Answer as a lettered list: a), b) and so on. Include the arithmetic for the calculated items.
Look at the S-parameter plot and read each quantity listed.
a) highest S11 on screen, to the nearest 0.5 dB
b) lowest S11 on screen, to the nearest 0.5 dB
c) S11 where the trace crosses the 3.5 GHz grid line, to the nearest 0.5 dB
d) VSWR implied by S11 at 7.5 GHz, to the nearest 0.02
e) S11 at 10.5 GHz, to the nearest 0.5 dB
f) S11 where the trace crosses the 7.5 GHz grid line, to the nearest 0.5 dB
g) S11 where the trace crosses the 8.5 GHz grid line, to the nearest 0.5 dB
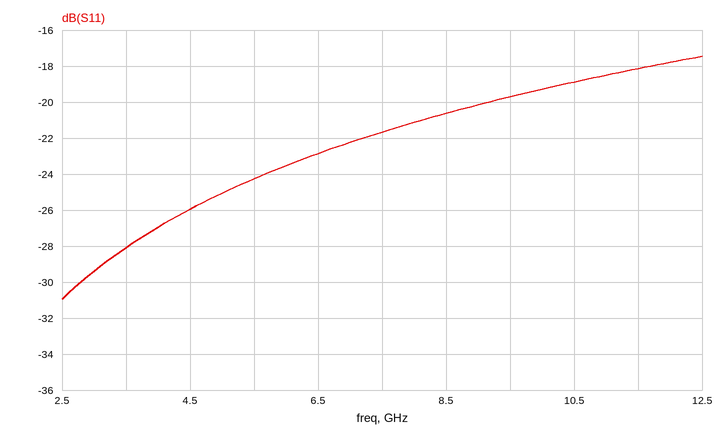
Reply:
a) -17.5 dB
b) -31.0 dB
c) -28.0 dB
d) |Γ| = 10^(-21.5/20) = 0.0841; VSWR = (1 + 0.0841)/(1 − 0.0841) ≈ 1.18
e) -19.0 dB
f) -21.5 dB
g) -20.5 dB
